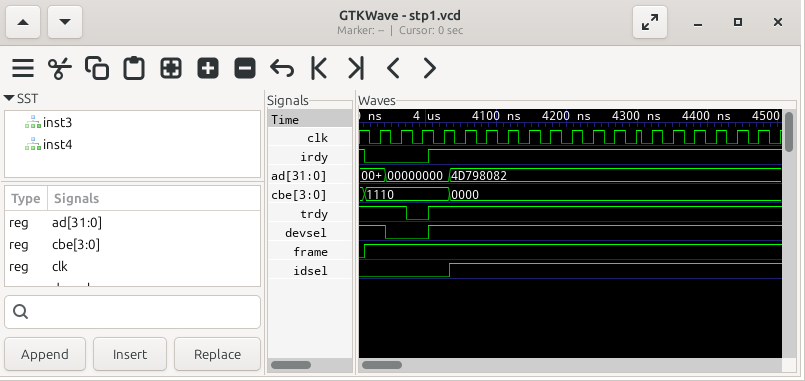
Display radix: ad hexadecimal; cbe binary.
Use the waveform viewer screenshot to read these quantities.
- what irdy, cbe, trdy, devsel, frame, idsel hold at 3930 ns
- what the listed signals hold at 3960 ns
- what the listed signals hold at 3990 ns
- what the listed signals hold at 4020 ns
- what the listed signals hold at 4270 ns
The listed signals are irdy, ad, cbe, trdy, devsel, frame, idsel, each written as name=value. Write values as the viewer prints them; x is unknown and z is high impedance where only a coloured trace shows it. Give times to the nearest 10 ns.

irdy=0, cbe=1110, trdy=1, devsel=1, frame=1, idsel=0
irdy=0, ad=00000000, cbe=1110, trdy=1, devsel=0, frame=1, idsel=0
irdy=0, ad=00000000, cbe=1110, trdy=0, devsel=0, frame=1, idsel=0
irdy=1, ad=00000000, cbe=1110, trdy=1, devsel=1, frame=1, idsel=0
irdy=1, ad=4D798082, cbe=0000, trdy=1, devsel=1, frame=1, idsel=1
